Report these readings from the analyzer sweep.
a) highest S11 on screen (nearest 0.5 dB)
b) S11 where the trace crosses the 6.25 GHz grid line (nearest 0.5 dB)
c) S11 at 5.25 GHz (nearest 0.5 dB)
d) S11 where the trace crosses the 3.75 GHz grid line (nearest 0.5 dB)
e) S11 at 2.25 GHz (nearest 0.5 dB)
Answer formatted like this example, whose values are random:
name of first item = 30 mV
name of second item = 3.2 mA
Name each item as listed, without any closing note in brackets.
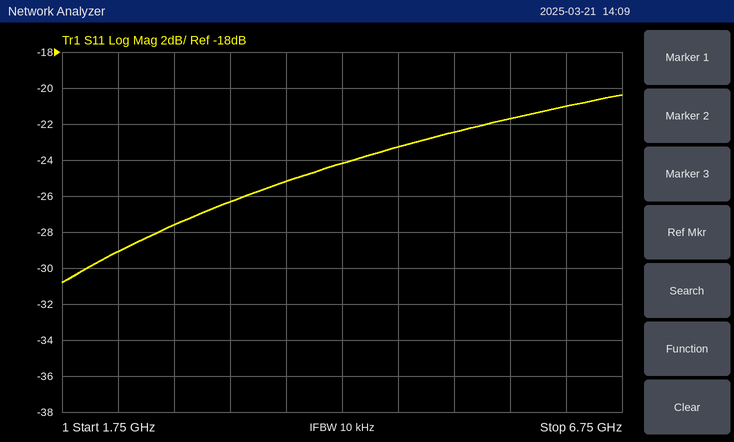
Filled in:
highest S11 on screen = -20.5 dB
S11 where the trace crosses the 6.25 GHz grid line = -21.0 dB
S11 at 5.25 GHz = -22.5 dB
S11 where the trace crosses the 3.75 GHz grid line = -25.0 dB
S11 at 2.25 GHz = -29.0 dB
